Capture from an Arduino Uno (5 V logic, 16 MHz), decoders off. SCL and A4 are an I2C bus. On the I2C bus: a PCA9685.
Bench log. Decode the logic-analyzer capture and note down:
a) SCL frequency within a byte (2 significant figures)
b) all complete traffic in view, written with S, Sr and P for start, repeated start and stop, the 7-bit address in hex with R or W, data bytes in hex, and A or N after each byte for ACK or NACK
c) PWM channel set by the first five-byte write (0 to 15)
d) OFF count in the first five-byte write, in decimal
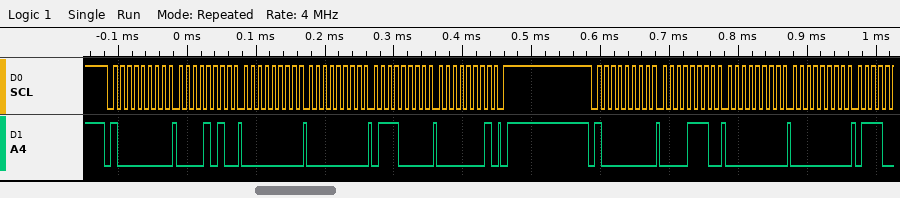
100 kHz
S 40W A 0A A 00 A 00 A 70 A 01 A P S 40W A 0E A 00 A 00 A
1
368
